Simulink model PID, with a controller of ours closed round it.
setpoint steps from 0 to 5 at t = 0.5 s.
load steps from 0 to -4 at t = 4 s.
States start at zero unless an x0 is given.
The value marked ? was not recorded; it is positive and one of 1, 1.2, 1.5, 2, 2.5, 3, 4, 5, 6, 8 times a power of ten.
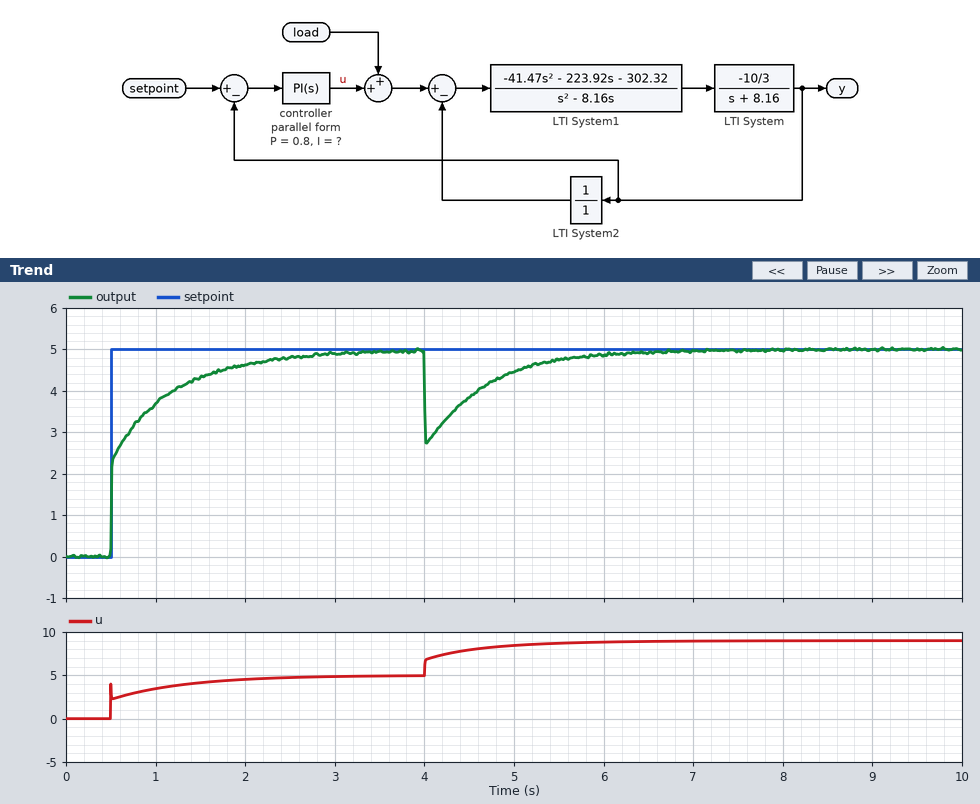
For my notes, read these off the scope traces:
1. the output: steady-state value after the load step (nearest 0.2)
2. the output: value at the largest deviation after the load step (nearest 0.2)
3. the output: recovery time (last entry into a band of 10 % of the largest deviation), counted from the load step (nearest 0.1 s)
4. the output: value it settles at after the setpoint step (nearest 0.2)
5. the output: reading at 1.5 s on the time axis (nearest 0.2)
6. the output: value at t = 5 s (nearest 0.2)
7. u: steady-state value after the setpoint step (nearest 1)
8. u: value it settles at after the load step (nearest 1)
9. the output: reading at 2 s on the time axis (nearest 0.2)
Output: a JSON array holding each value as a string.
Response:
["5.0", "2.8", "1.6 s", "5.0", "4.4", "4.4", "5", "9", "4.6"]
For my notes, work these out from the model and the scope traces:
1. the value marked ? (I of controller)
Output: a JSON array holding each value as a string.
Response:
["2.5"]
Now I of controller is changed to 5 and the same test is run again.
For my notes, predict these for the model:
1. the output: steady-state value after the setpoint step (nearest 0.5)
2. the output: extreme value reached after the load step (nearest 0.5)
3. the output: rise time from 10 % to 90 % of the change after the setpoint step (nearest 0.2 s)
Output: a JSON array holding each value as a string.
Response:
["5.0", "3.0", "0.6 s"]
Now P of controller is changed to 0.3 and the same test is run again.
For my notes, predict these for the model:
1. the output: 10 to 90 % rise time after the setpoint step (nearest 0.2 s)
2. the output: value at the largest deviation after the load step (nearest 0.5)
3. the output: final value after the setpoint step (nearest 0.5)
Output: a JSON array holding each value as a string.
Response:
["1.0 s", "2.0", "5.0"]
